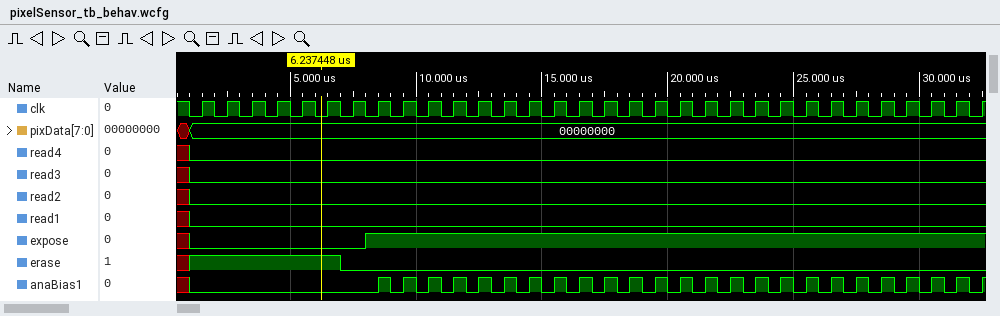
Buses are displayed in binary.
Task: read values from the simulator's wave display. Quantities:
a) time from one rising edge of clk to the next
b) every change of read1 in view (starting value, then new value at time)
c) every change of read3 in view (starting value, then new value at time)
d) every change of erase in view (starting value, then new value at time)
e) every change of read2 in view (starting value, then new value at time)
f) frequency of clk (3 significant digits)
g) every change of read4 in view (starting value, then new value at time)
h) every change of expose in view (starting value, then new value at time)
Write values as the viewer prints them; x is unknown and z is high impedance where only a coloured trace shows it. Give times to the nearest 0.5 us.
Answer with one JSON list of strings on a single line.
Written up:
["1 us", "x, 0 at 1 us", "x, 0 at 1 us", "x, 1 at 1 us, 0 at 7 us", "x, 0 at 1 us", "1.00 MHz", "x, 0 at 1 us", "x, 0 at 1 us, 1 at 8 us"]
